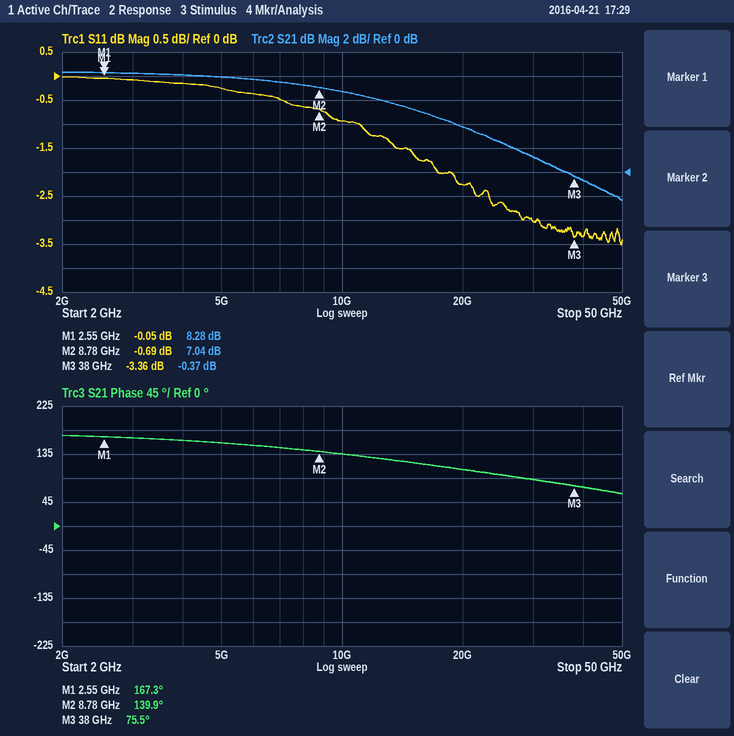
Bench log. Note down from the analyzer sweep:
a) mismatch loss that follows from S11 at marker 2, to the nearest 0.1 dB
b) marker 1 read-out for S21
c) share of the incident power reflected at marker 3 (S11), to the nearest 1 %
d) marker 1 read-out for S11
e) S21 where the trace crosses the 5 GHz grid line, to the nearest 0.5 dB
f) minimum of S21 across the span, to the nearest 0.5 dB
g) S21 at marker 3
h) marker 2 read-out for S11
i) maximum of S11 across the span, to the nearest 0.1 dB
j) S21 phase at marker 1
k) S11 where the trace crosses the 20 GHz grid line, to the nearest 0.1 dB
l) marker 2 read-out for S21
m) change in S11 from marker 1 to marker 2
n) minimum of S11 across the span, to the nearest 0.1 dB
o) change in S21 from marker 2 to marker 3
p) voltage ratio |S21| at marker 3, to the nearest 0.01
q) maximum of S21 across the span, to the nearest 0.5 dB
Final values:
8.3 dB
8.28 dB
46 %
-0.05 dB
8.0 dB
-2.5 dB
-0.37 dB
-0.69 dB
0.0 dB
167.3°
-2.3 dB
7.04 dB
-0.64 dB
-3.5 dB
-7.41 dB
0.96
8.5 dB
